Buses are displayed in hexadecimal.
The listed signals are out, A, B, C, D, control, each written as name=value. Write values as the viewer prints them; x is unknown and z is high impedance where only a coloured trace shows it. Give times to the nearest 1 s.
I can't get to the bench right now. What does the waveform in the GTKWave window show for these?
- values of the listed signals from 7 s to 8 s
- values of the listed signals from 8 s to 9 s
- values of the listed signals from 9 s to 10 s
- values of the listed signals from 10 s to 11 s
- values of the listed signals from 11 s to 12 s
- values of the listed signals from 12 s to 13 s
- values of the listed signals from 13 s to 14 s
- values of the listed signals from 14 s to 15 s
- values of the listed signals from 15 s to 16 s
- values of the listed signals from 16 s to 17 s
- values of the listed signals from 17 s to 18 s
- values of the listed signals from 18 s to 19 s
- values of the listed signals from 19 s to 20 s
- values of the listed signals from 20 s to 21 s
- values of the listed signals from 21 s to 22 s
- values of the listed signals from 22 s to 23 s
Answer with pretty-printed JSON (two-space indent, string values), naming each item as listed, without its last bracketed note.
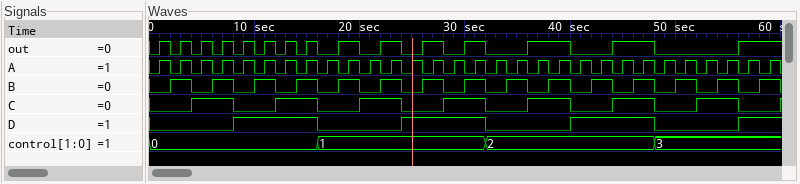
{
  "values of the listed signals from 7 s to 8 s": "out=1, A=1, B=1, C=1, D=0, control=0",
  "values of the listed signals from 8 s to 9 s": "out=0, A=0, B=0, C=0, D=1, control=0",
  "values of the listed signals from 9 s to 10 s": "out=1, A=1, B=0, C=0, D=1, control=0",
  "values of the listed signals from 10 s to 11 s": "out=0, A=0, B=1, C=0, D=1, control=0",
  "values of the listed signals from 11 s to 12 s": "out=1, A=1, B=1, C=0, D=1, control=0",
  "values of the listed signals from 12 s to 13 s": "out=0, A=0, B=0, C=1, D=1, control=0",
  "values of the listed signals from 13 s to 14 s": "out=1, A=1, B=0, C=1, D=1, control=0",
  "values of the listed signals from 14 s to 15 s": "out=0, A=0, B=1, C=1, D=1, control=0",
  "values of the listed signals from 15 s to 16 s": "out=1, A=1, B=1, C=1, D=1, control=0",
  "values of the listed signals from 16 s to 17 s": "out=0, A=0, B=0, C=0, D=0, control=1",
  "values of the listed signals from 17 s to 18 s": "out=0, A=1, B=0, C=0, D=0, control=1",
  "values of the listed signals from 18 s to 19 s": "out=1, A=0, B=1, C=0, D=0, control=1",
  "values of the listed signals from 19 s to 20 s": "out=1, A=1, B=1, C=0, D=0, control=1",
  "values of the listed signals from 20 s to 21 s": "out=0, A=0, B=0, C=1, D=0, control=1",
  "values of the listed signals from 21 s to 22 s": "out=0, A=1, B=0, C=1, D=0, control=1",
  "values of the listed signals from 22 s to 23 s": "out=1, A=0, B=1, C=1, D=0, control=1"
}
